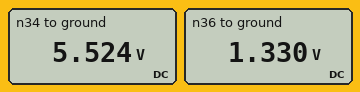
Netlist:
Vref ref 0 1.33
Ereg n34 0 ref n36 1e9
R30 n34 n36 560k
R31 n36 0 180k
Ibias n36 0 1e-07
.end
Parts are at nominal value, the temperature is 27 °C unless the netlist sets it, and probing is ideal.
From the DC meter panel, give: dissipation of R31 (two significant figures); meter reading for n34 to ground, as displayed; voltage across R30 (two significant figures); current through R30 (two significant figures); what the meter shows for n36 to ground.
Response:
9.8 µW
5.524 V
4.2 V
7.5 µA
1.330 V
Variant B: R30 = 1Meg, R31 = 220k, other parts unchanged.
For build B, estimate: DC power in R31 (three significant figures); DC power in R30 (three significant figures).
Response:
8.04 µW
37.8 µW
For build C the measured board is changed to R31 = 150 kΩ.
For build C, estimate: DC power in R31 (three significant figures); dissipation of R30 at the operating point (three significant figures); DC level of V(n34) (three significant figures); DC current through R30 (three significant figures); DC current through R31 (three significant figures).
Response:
11.8 µW
45.0 µW
6.35 V
8.97 µA
8.87 µA
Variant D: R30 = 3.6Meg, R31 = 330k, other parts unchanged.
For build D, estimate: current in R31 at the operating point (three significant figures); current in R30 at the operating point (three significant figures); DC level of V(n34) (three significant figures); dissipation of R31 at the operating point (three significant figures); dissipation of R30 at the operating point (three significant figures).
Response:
4.03 µA
4.13 µA
16.2 V
5.36 µW
61.4 µW
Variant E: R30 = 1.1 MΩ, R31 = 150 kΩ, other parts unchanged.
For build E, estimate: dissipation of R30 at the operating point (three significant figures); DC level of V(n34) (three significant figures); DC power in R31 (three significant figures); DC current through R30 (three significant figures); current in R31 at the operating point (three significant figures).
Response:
88.4 µW
11.2 V
11.8 µW
8.97 µA
8.87 µA
